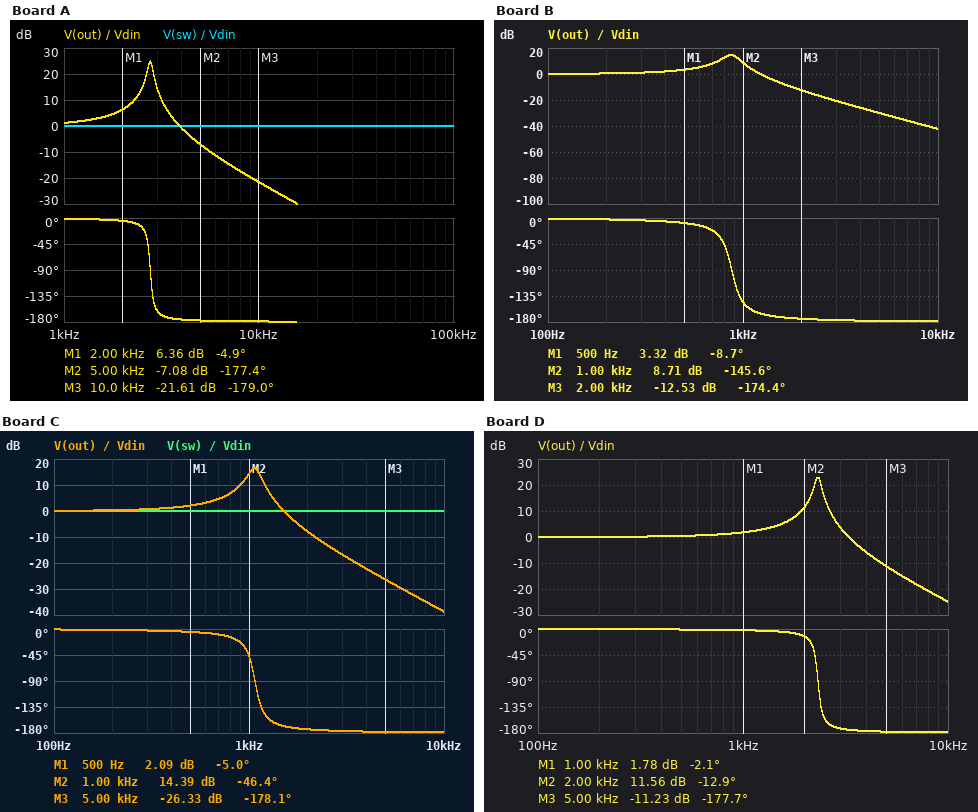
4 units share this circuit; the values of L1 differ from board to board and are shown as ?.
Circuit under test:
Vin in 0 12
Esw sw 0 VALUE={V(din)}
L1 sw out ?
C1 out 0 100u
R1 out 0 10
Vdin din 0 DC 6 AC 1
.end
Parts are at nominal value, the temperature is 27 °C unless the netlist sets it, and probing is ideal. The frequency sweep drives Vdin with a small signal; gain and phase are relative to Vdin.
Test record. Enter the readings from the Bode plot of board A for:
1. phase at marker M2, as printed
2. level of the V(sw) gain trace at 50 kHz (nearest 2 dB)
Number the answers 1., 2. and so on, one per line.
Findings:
1. -177.4 deg
2. 0 dB
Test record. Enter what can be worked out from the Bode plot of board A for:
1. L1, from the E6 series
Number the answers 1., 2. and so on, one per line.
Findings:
1. 33 µH
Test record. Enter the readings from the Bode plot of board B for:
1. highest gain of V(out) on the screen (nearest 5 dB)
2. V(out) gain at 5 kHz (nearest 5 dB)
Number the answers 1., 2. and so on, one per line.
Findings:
1. 15 dB
2. -30 dB
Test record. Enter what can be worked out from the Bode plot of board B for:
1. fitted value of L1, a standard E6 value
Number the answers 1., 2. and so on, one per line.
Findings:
1. 330 µH
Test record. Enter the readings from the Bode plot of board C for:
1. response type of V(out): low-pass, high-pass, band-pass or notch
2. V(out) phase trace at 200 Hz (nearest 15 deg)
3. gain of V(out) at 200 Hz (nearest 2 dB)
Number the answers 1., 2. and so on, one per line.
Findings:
1. low-pass
2. 0 deg
3. 0 dB
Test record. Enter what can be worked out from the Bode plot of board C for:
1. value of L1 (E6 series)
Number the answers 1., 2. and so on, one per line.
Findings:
1. 220 µH
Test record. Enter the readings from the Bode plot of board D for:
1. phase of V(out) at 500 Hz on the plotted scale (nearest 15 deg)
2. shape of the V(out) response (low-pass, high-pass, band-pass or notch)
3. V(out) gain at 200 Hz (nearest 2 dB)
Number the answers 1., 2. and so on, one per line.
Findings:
1. 0 deg
2. low-pass
3. 0 dB
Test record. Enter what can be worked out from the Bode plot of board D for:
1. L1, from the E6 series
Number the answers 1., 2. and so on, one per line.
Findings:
1. 47 µH
